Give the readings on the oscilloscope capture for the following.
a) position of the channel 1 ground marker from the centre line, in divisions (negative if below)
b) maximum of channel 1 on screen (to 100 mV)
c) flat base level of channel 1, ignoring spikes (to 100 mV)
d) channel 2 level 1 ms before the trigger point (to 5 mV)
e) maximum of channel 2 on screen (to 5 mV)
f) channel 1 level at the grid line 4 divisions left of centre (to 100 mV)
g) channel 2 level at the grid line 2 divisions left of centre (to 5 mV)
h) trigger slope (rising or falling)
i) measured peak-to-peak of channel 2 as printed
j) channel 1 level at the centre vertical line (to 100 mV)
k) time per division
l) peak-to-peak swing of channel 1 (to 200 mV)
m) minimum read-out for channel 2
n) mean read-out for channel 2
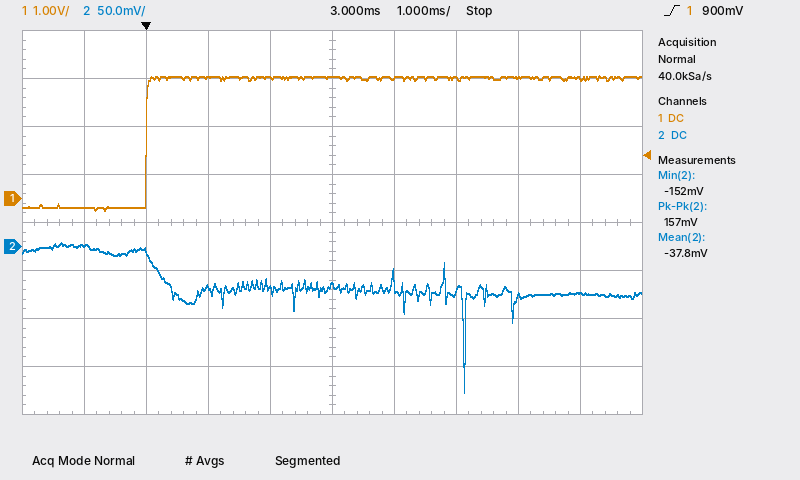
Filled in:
+0.5 div
2.6 V
-200 mV
0 mV
5 mV
-200 mV
-45 mV
rising
157 mV
2.5 V
1 ms
2.8 V
-152 mV
-37.8 mV
